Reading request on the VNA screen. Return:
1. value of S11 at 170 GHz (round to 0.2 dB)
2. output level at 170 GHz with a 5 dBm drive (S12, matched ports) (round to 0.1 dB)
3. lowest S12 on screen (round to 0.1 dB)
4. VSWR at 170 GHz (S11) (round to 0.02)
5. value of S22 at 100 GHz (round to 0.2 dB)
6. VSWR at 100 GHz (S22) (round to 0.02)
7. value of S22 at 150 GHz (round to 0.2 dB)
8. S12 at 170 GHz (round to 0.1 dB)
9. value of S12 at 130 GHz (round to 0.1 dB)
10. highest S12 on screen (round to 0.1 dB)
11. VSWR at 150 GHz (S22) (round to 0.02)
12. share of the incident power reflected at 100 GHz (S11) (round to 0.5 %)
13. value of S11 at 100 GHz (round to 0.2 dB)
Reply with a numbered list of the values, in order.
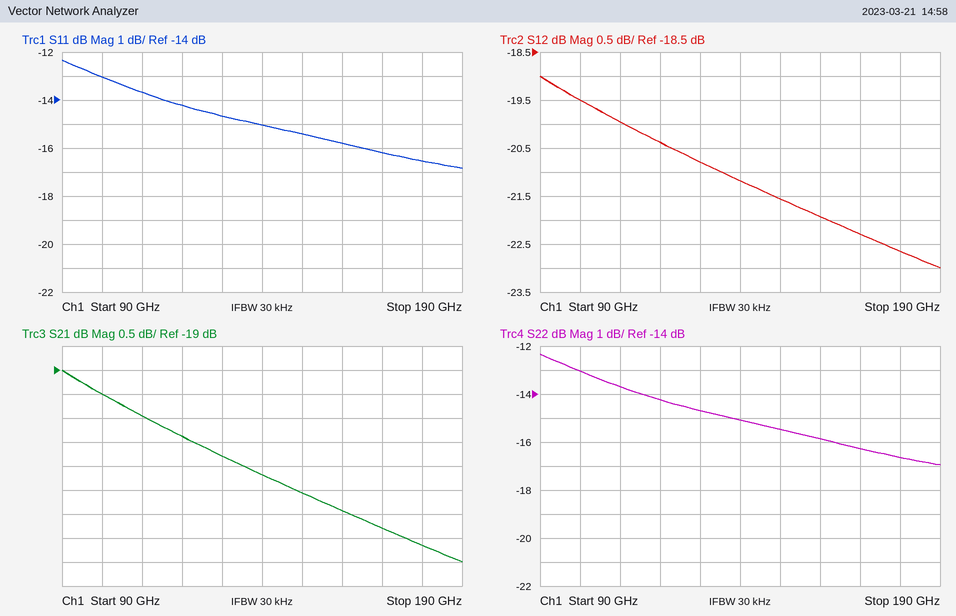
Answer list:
1. -16.2 dB
2. -17.3 dBm
3. -23.0 dB
4. 1.36
5. -13.0 dB
6. 1.58
7. -15.4 dB
8. -22.3 dB
9. -20.8 dB
10. -19.0 dB
11. 1.40
12. 5.0 %
13. -13.0 dB
